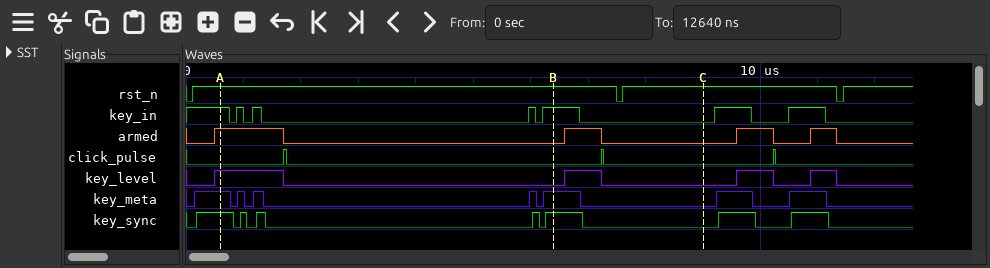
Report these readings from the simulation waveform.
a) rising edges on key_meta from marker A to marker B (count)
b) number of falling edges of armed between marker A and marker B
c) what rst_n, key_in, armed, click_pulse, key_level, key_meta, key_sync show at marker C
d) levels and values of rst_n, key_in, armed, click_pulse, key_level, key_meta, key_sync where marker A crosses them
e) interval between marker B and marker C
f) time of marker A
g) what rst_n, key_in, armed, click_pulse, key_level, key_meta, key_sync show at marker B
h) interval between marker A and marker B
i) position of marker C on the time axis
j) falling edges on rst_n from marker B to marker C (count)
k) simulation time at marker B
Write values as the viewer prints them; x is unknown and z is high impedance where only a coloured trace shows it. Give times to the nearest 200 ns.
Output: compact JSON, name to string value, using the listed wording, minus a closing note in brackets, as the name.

{"rising edges on key_meta from marker A to marker B": "4", "number of falling edges of armed between marker A and marker B": "1", "what rst_n, key_in, armed, click_pulse, key_level, key_meta, key_sync show at marker C": "rst_n=1, key_in=0, armed=0, click_pulse=0, key_level=0, key_meta=0, key_sync=0", "levels and values of rst_n, key_in, armed, click_pulse, key_level, key_meta, key_sync where marker A crosses them": "rst_n=1, key_in=1, armed=1, click_pulse=0, key_level=1, key_meta=1, key_sync=1", "interval between marker B and marker C": "2600 ns", "time of marker A": "600 ns", "what rst_n, key_in, armed, click_pulse, key_level, key_meta, key_sync show at marker B": "rst_n=1, key_in=1, armed=0, click_pulse=0, key_level=0, key_meta=1, key_sync=1", "interval between marker A and marker B": "5800 ns", "position of marker C on the time axis": "9000 ns", "falling edges on rst_n from marker B to marker C": "1", "simulation time at marker B": "6400 ns"}
